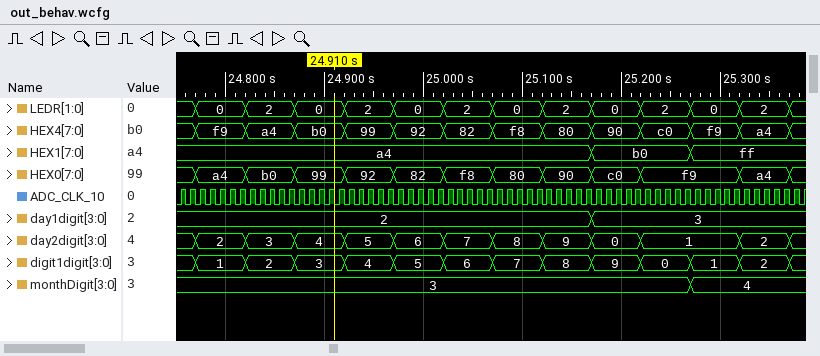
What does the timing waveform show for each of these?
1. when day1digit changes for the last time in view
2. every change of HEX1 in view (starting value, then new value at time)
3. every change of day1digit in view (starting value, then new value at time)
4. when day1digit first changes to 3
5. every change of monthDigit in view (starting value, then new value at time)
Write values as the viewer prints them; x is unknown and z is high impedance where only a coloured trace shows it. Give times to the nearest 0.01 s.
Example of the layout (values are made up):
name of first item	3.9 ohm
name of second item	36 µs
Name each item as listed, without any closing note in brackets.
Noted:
when day1digit changes for the last time in view	25.17 s
every change of HEX1 in view	a4, b0 at 25.17 s, ff at 25.27 s
every change of day1digit in view	2, 3 at 25.17 s
when day1digit first changes to 3	25.17 s
every change of monthDigit in view	3, 4 at 25.27 s
